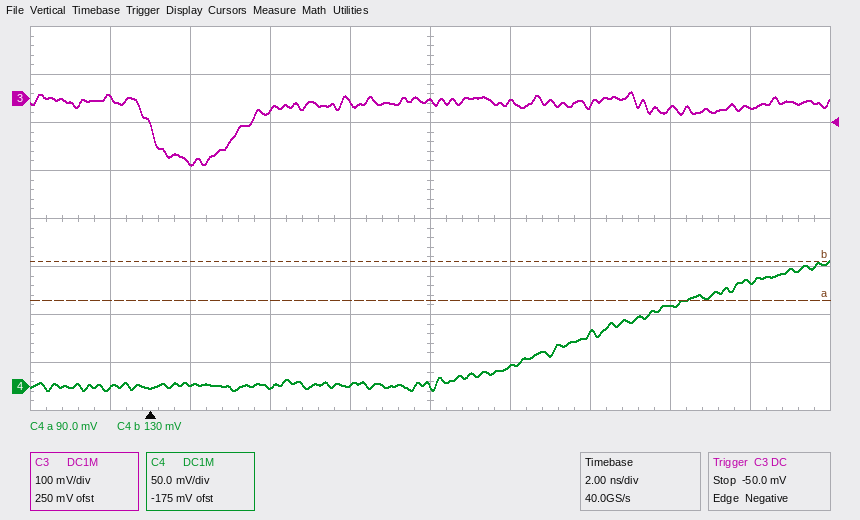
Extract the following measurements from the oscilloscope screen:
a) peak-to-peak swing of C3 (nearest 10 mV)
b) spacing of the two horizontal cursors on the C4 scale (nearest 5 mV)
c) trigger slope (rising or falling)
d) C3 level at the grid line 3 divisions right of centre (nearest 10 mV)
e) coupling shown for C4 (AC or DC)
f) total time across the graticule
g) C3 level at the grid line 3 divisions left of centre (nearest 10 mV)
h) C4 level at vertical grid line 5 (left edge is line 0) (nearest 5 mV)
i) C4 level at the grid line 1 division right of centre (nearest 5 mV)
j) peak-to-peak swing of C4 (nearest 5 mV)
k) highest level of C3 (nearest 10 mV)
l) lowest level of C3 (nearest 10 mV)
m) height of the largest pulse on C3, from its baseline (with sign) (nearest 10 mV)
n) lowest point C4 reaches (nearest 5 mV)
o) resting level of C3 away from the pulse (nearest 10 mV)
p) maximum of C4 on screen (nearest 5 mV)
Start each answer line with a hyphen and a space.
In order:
- 150 mV
- 40 mV
- falling
- -20 mV
- DC
- 20 ns
- -130 mV
- 0 mV
- 20 mV
- 135 mV
- 10 mV
- -140 mV
- -130 mV
- -5 mV
- -10 mV
- 130 mV
